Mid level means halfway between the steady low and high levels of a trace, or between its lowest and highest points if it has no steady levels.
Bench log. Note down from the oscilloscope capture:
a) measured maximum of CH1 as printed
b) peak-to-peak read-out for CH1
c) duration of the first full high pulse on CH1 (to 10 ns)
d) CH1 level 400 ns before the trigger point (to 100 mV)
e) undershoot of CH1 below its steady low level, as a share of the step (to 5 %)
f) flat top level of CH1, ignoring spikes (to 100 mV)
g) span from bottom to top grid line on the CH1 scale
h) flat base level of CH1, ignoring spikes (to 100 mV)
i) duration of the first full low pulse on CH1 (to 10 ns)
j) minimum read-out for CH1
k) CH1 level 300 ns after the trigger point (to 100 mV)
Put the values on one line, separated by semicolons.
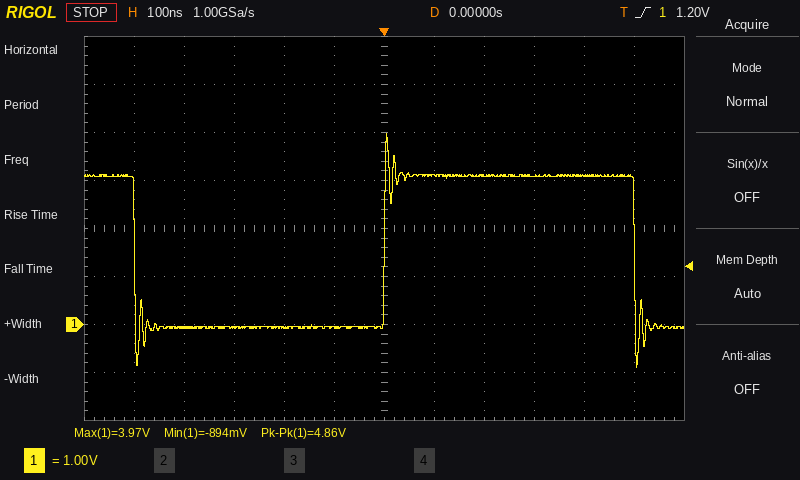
3.97 V; 4.86 V; 500 ns; -100 mV; 25 %; 3.1 V; 8 V; -100 mV; 500 ns; -894 mV; 3.1 V
